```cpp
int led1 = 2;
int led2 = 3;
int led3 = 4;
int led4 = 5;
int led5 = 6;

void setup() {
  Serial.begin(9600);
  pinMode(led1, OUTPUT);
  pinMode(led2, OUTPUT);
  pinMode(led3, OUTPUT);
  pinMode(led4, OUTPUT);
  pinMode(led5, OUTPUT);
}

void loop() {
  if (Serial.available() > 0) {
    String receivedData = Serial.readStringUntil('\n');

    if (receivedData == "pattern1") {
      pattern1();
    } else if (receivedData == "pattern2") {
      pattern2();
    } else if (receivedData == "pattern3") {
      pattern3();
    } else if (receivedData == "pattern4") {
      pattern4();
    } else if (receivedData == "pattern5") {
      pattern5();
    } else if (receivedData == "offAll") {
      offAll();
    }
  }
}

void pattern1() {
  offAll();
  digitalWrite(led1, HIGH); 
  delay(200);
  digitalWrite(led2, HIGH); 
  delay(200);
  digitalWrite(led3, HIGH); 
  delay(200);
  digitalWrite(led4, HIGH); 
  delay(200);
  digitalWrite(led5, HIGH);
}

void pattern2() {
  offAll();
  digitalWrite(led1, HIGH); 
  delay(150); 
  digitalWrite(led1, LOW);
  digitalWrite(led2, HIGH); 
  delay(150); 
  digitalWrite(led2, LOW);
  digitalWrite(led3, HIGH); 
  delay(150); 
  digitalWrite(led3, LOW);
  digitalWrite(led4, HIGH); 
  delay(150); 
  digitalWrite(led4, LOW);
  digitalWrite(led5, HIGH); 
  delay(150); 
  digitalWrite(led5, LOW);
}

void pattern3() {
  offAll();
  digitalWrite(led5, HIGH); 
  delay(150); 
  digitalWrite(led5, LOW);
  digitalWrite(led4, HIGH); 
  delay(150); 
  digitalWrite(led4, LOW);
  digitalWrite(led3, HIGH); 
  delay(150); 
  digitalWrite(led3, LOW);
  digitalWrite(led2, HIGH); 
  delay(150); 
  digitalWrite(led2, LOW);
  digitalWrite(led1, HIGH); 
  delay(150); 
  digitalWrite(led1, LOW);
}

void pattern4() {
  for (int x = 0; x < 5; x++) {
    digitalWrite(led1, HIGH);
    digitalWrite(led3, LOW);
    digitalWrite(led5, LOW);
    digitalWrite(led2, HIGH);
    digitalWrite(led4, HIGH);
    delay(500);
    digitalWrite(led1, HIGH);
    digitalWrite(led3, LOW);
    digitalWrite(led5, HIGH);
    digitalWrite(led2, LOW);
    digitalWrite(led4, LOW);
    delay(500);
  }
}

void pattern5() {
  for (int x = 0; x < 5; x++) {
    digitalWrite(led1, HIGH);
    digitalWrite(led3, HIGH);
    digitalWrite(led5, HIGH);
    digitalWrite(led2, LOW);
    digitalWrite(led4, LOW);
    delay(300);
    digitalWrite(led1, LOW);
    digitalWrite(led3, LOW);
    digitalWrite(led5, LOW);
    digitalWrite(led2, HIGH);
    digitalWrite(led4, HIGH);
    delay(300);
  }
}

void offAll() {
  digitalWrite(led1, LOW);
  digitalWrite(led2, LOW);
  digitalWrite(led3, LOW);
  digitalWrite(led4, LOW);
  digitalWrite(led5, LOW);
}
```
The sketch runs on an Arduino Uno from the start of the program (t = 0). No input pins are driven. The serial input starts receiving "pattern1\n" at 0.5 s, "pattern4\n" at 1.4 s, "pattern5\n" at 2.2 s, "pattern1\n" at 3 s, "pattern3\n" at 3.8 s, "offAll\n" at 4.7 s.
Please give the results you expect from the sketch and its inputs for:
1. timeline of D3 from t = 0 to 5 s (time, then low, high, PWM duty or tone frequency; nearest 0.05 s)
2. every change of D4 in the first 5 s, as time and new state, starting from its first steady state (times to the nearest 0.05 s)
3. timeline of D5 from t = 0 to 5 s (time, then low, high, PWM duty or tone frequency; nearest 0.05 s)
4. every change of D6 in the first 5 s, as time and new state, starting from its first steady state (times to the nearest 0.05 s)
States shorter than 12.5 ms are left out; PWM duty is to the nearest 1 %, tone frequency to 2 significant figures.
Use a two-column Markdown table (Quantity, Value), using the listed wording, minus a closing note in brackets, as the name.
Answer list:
| Quantity | Value |
|---|---|
| timeline of D3 from t = 0 to 5 s | 0 s low; 0.7 s high; 1.9 s low; 2.4 s high; 2.9 s low; 3.4 s high; 3.9 s low; 4.4 s high; 4.9 s low |
| every change of D4 in the first 5 s, as time and new state, starting from its first steady state | 0 s low; 0.9 s high; 1.4 s low |
| timeline of D5 from t = 0 to 5 s | 0 s low; 1.1 s high; 1.9 s low; 2.4 s high; 2.9 s low; 3.4 s high; 3.9 s low; 4.4 s high; 4.9 s low |
| every change of D6 in the first 5 s, as time and new state, starting from its first steady state | 0 s low; 1.3 s high; 1.4 s low; 1.9 s high; 2.4 s low; 2.9 s high; 3.4 s low; 3.9 s high; 4.4 s low; 4.9 s high |
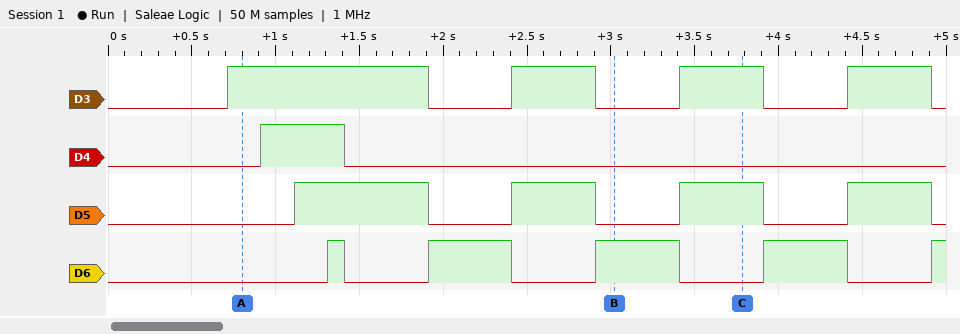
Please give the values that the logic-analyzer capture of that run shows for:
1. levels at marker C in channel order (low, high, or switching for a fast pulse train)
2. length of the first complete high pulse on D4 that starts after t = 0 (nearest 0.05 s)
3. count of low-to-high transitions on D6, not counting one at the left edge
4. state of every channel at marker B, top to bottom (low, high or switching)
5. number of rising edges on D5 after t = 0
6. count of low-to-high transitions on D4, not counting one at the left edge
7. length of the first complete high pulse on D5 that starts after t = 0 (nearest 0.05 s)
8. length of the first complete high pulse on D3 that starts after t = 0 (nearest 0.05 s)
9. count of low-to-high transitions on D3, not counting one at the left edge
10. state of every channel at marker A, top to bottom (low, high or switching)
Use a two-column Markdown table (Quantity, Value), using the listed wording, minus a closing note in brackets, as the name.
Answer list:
| Quantity | Value |
|---|---|
| levels at marker C in channel order | D3 high, D4 low, D5 high, D6 low |
| length of the first complete high pulse on D4 that starts after t = 0 | 0.50 s |
| count of low-to-high transitions on D6, not counting one at the left edge | 5 |
| state of every channel at marker B, top to bottom | D3 low, D4 low, D5 low, D6 high |
| number of rising edges on D5 after t = 0 | 4 |
| count of low-to-high transitions on D4, not counting one at the left edge | 1 |
| length of the first complete high pulse on D5 that starts after t = 0 | 0.80 s |
| length of the first complete high pulse on D3 that starts after t = 0 | 1.20 s |
| count of low-to-high transitions on D3, not counting one at the left edge | 4 |
| state of every channel at marker A, top to bottom | D3 high, D4 low, D5 low, D6 low |
